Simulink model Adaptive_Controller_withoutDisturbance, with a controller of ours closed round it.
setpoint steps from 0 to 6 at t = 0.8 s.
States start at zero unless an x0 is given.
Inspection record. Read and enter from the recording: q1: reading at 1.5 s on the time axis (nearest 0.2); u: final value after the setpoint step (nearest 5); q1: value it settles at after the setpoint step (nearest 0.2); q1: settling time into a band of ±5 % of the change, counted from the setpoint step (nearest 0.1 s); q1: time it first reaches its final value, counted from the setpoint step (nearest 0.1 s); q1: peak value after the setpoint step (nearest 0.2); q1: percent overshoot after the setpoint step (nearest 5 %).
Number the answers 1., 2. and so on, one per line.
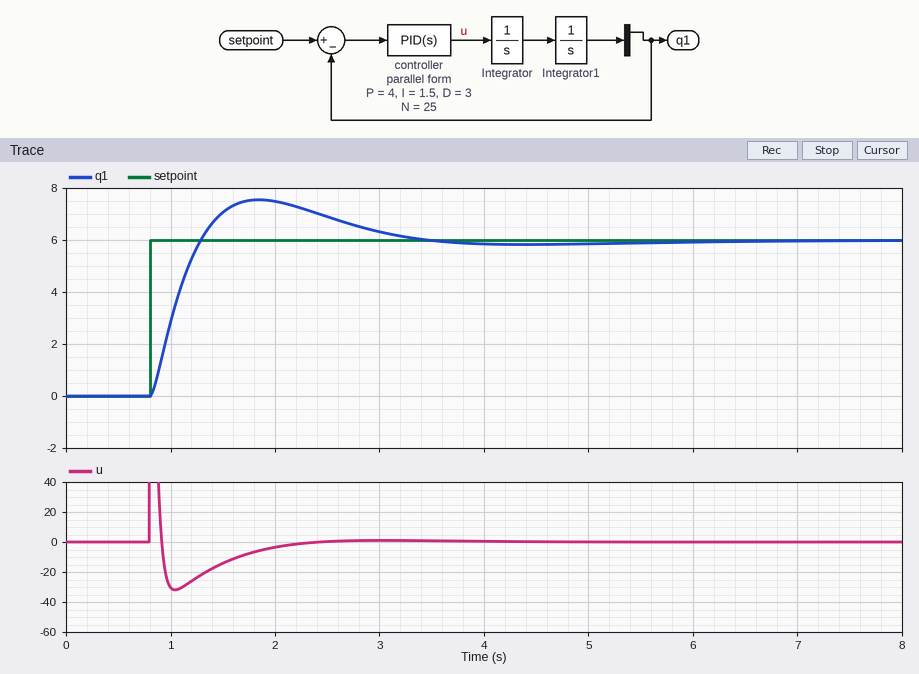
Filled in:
1. 7.0
2. 0
3. 6.0
4. 2.2 s
5. 0.5 s
6. 7.6
7. 25 %
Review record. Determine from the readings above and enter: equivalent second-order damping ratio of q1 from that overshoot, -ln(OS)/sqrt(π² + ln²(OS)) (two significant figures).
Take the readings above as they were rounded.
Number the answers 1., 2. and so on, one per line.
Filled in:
1. 0.40
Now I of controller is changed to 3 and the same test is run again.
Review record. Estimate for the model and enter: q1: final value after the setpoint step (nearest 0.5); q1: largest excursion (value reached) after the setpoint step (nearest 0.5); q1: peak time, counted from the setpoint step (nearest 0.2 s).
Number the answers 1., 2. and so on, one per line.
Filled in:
1. 6.0
2. 8.0
3. 1.0 s
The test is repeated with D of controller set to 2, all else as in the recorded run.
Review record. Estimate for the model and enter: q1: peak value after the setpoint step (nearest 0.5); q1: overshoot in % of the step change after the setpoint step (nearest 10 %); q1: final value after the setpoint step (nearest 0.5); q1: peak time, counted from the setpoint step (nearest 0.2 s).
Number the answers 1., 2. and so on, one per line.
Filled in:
1. 8.5
2. 40 %
3. 6.0
4. 1.2 s
